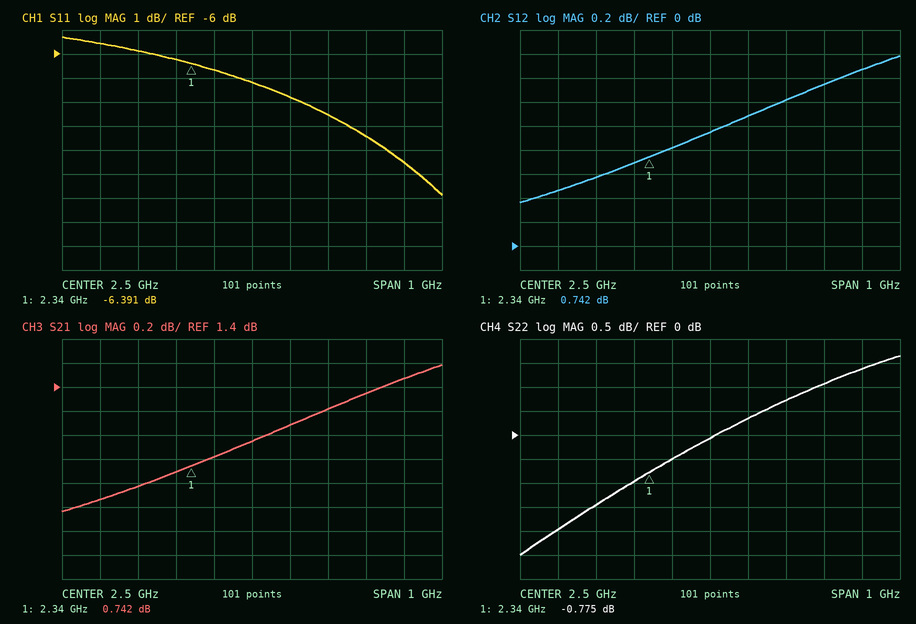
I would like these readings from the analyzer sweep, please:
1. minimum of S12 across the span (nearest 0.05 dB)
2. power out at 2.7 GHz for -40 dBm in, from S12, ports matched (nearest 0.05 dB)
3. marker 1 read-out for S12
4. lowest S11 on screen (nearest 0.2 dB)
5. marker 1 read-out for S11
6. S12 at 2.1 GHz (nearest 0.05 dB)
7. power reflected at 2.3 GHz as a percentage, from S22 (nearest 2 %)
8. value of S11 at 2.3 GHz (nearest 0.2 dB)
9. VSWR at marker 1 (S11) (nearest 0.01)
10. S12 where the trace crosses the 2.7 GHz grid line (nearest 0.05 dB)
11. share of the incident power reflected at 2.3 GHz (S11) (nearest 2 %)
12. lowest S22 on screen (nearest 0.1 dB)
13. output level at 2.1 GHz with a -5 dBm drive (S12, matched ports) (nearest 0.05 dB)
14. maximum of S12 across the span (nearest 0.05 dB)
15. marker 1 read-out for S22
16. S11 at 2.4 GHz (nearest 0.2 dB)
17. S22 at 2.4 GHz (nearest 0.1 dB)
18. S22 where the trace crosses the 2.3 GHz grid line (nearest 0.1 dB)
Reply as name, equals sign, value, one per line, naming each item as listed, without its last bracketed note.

minimum of S12 across the span = 0.35 dB
power out at 2.7 GHz for -40 dBm in, from S12, ports matched = -38.80 dBm
marker 1 read-out for S12 = 0.742 dB
lowest S11 on screen = -11.8 dB
marker 1 read-out for S11 = -6.391 dB
S12 at 2.1 GHz = 0.45 dB
power reflected at 2.3 GHz as a percentage, from S22 = 80 %
value of S11 at 2.3 GHz = -6.2 dB
VSWR at marker 1 (S11) = 2.84
S12 where the trace crosses the 2.7 GHz grid line = 1.20 dB
share of the incident power reflected at 2.3 GHz (S11) = 24 %
lowest S22 on screen = -2.5 dB
output level at 2.1 GHz with a -5 dBm drive (S12, matched ports) = -4.55 dBm
maximum of S12 across the span = 1.60 dB
marker 1 read-out for S22 = -0.775 dB
S11 at 2.4 GHz = -6.6 dB
S22 at 2.4 GHz = -0.5 dB
S22 where the trace crosses the 2.3 GHz grid line = -1.0 dB
